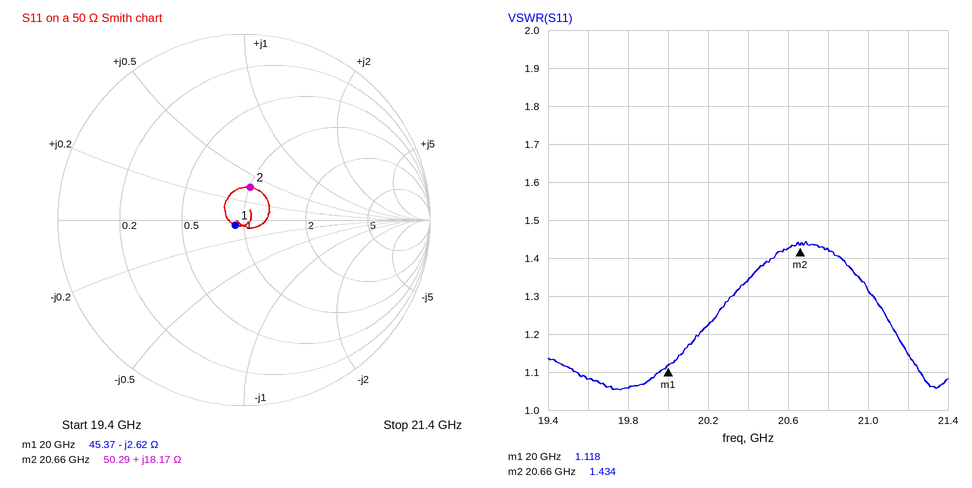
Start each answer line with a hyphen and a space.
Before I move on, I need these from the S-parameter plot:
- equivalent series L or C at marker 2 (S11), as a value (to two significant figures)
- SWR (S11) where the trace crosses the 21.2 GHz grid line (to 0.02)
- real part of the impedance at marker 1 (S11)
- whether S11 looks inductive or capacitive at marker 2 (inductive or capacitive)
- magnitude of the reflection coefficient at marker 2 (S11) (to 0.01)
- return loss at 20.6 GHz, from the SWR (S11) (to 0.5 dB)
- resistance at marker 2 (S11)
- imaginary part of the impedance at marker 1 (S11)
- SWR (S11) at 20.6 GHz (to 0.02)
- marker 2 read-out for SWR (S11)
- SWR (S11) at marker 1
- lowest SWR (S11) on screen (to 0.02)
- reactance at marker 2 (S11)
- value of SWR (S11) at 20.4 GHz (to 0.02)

- 140 pH
- 1.14
- 45.37 Ω
- inductive
- 0.18
- 15.0 dB
- 50.29 Ω
- -2.62 Ω
- 1.42
- 1.434
- 1.118
- 1.06
- +18.17 Ω
- 1.34
